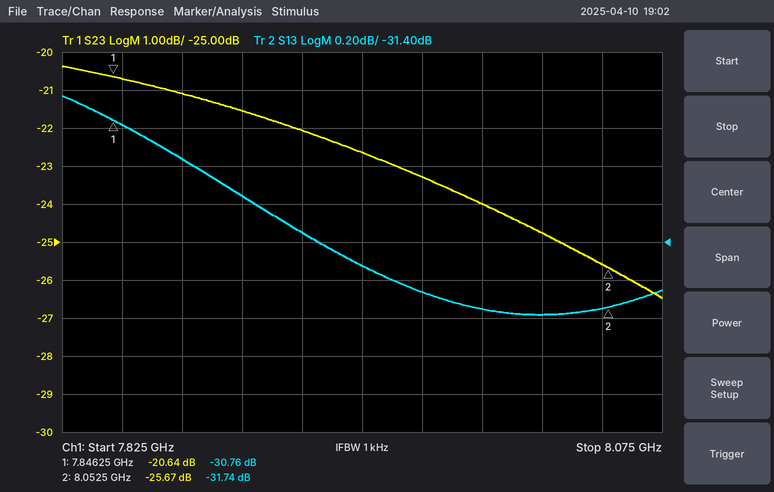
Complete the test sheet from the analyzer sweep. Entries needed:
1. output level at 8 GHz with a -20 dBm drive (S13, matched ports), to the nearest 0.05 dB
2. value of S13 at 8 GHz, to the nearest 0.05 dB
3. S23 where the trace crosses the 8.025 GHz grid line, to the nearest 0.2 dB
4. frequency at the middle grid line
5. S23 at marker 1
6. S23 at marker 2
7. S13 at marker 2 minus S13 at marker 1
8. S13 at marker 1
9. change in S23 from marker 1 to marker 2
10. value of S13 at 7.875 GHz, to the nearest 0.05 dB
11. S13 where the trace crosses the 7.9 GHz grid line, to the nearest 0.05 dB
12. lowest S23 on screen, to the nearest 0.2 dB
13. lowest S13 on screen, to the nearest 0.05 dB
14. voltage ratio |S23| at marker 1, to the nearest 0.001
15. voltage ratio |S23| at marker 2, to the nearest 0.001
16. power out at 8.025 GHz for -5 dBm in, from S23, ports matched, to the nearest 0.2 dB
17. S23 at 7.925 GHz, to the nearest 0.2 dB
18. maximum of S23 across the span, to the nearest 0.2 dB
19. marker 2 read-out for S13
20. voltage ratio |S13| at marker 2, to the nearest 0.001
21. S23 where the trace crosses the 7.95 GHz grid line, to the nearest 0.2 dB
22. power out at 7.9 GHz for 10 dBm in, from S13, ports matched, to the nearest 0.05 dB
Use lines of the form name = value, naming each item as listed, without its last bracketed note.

output level at 8 GHz with a -20 dBm drive (S13, matched ports), to the nearest 0.05 dB = -51.75 dBm
value of S13 at 8 GHz, to the nearest 0.05 dB = -31.75 dB
S23 where the trace crosses the 8.025 GHz grid line, to the nearest 0.2 dB = -24.8 dB
frequency at the middle grid line = 7.95 GHz
S23 at marker 1 = -20.64 dB
S23 at marker 2 = -25.67 dB
S13 at marker 2 minus S13 at marker 1 = -0.98 dB
S13 at marker 1 = -30.76 dB
change in S23 from marker 1 to marker 2 = -5.03 dB
value of S13 at 7.875 GHz, to the nearest 0.05 dB = -30.95 dB
S13 where the trace crosses the 7.9 GHz grid line, to the nearest 0.05 dB = -31.15 dB
lowest S23 on screen, to the nearest 0.2 dB = -26.4 dB
lowest S13 on screen, to the nearest 0.05 dB = -31.80 dB
voltage ratio |S23| at marker 1, to the nearest 0.001 = 0.093
voltage ratio |S23| at marker 2, to the nearest 0.001 = 0.052
power out at 8.025 GHz for -5 dBm in, from S23, ports matched, to the nearest 0.2 dB = -29.8 dBm
S23 at 7.925 GHz, to the nearest 0.2 dB = -22.0 dB
maximum of S23 across the span, to the nearest 0.2 dB = -20.4 dB
marker 2 read-out for S13 = -31.74 dB
voltage ratio |S13| at marker 2, to the nearest 0.001 = 0.026
S23 where the trace crosses the 7.95 GHz grid line, to the nearest 0.2 dB = -22.6 dB
power out at 7.9 GHz for 10 dBm in, from S13, ports matched, to the nearest 0.05 dB = -21.15 dBm
